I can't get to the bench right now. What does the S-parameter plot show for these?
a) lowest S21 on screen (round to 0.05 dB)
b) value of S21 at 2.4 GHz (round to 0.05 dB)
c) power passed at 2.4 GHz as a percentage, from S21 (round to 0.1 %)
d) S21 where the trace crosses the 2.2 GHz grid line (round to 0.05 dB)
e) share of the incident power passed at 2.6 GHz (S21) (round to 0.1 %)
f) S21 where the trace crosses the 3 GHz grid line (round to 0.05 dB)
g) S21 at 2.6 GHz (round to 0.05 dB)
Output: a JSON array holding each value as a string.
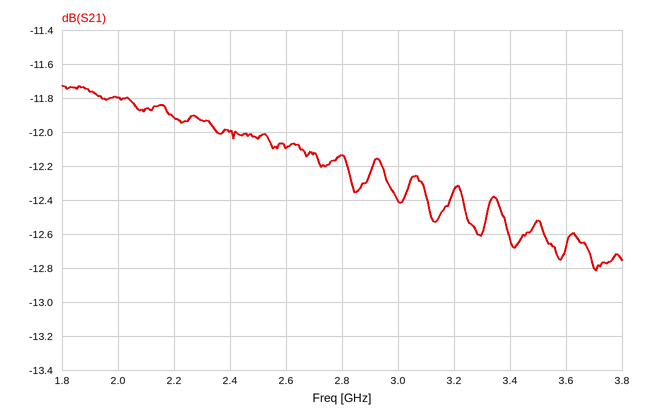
["-12.80 dB", "-12.00 dB", "6.3 %", "-11.90 dB", "6.2 %", "-12.40 dB", "-12.10 dB"]
